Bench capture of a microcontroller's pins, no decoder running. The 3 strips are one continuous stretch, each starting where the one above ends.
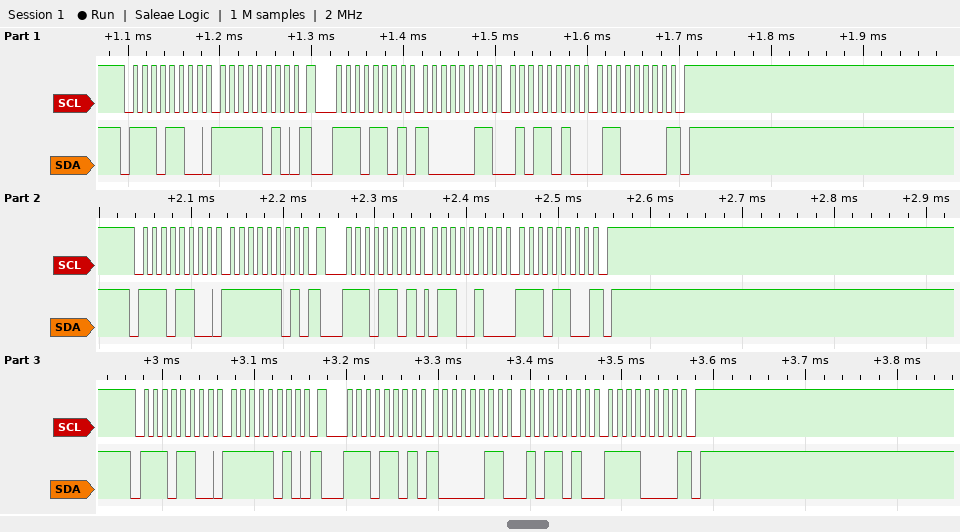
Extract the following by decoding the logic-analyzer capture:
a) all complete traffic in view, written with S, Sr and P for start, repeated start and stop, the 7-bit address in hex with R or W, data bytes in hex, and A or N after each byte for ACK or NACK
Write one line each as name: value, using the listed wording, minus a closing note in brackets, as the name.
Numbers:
all complete traffic in view, written with S, Sr and P for start, repeated start and stop, the 7-bit address in hex with R or W, data bytes in hex, and A or N after each byte for ACK or NACK: S 76W A FA A Sr 76R A 83 A 5A A 60 N P S 76W A FD A Sr 76R A 64 A EC N P S 76W A FA A Sr 76R A 83 A 5A A F0 N P
